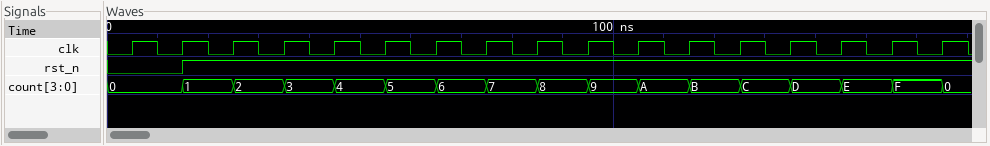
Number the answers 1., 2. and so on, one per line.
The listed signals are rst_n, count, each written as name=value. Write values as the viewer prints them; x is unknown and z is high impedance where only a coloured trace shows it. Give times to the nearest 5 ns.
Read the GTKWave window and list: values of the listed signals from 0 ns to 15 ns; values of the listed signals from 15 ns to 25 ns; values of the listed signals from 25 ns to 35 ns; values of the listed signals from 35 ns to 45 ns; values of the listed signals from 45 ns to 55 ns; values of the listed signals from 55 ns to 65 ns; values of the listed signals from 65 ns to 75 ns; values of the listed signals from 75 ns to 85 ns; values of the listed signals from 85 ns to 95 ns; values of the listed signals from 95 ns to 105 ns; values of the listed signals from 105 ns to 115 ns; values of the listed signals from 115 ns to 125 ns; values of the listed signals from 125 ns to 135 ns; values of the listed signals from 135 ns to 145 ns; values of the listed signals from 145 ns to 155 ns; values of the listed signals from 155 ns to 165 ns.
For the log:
1. rst_n=0, count=0
2. rst_n=1, count=1
3. rst_n=1, count=2
4. rst_n=1, count=3
5. rst_n=1, count=4
6. rst_n=1, count=5
7. rst_n=1, count=6
8. rst_n=1, count=7
9. rst_n=1, count=8
10. rst_n=1, count=9
11. rst_n=1, count=A
12. rst_n=1, count=B
13. rst_n=1, count=C
14. rst_n=1, count=D
15. rst_n=1, count=E
16. rst_n=1, count=F
